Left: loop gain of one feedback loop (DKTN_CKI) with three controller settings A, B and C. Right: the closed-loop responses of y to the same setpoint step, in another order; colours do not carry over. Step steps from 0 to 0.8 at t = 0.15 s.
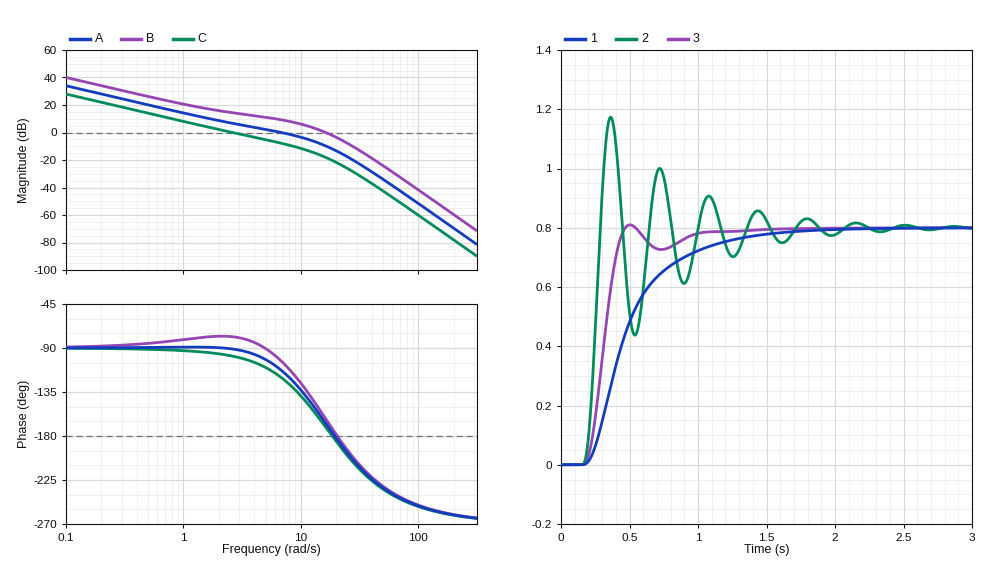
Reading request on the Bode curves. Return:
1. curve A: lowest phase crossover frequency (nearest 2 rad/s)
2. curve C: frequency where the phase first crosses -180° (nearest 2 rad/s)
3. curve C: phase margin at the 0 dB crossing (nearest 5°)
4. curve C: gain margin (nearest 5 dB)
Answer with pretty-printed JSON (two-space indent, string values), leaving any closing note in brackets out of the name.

{
  "curve A: lowest phase crossover frequency": "20 rad/s",
  "curve C: frequency where the phase first crosses -180°": "18 rad/s",
  "curve C: phase margin at the 0 dB crossing": "80°",
  "curve C: gain margin": "20 dB"
}
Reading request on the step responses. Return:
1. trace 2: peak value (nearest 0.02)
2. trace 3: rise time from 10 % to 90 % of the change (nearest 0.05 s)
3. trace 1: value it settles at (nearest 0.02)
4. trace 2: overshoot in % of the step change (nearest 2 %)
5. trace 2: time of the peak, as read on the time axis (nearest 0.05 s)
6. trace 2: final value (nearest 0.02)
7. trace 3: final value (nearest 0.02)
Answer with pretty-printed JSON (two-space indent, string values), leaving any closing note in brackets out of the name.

{
  "trace 2: peak value": "1.18",
  "trace 3: rise time from 10 % to 90 % of the change": "0.20 s",
  "trace 1: value it settles at": "0.80",
  "trace 2: overshoot in % of the step change": "46 %",
  "trace 2: time of the peak, as read on the time axis": "0.35 s",
  "trace 2: final value": "0.80",
  "trace 3: final value": "0.80"
}
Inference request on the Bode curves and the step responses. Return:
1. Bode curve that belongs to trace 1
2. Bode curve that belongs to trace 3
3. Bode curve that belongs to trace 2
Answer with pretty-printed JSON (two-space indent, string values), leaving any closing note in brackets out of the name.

{
  "Bode curve that belongs to trace 1": "C",
  "Bode curve that belongs to trace 3": "A",
  "Bode curve that belongs to trace 2": "B"
}
